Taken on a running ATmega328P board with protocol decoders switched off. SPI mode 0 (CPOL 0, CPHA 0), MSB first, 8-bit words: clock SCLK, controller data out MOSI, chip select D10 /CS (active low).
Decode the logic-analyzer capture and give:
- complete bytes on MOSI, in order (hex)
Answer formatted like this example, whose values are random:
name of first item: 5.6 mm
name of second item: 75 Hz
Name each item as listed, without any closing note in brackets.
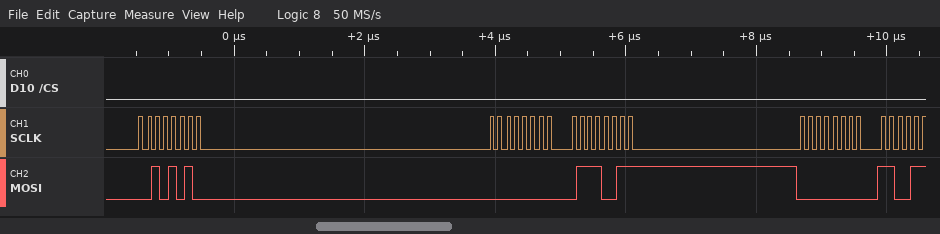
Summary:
complete bytes on MOSI, in order: 2A 00 73 00
